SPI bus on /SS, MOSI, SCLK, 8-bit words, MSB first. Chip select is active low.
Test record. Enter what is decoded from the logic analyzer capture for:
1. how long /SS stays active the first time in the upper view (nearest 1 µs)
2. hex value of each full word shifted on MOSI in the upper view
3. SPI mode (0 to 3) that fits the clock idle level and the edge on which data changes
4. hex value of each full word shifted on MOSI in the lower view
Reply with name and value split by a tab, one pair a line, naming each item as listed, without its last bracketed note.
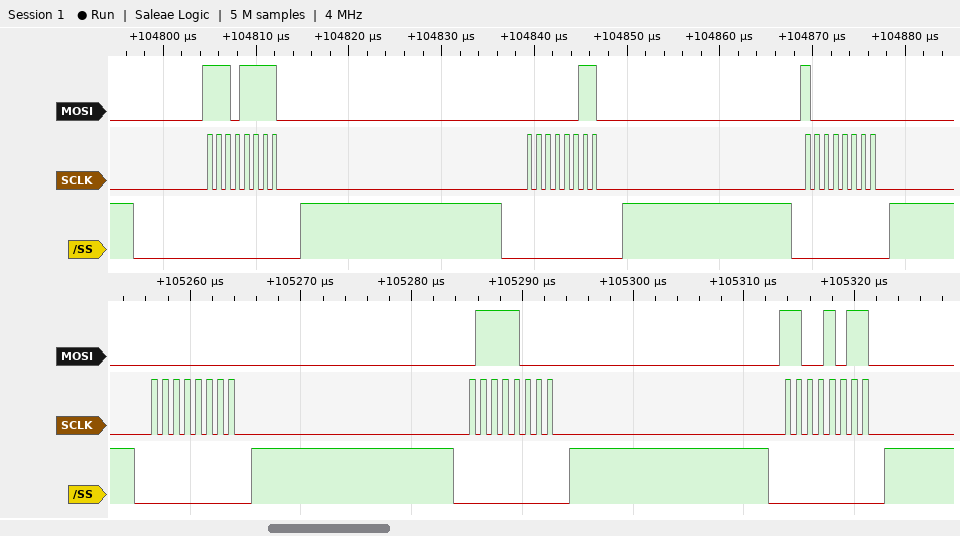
how long /SS stays active the first time in the upper view	18 µs
hex value of each full word shifted on MOSI in the upper view	EF, 03, 80
SPI mode (0 to 3) that fits the clock idle level and the edge on which data changes	0
hex value of each full word shifted on MOSI in the lower view	00, 78, CB
